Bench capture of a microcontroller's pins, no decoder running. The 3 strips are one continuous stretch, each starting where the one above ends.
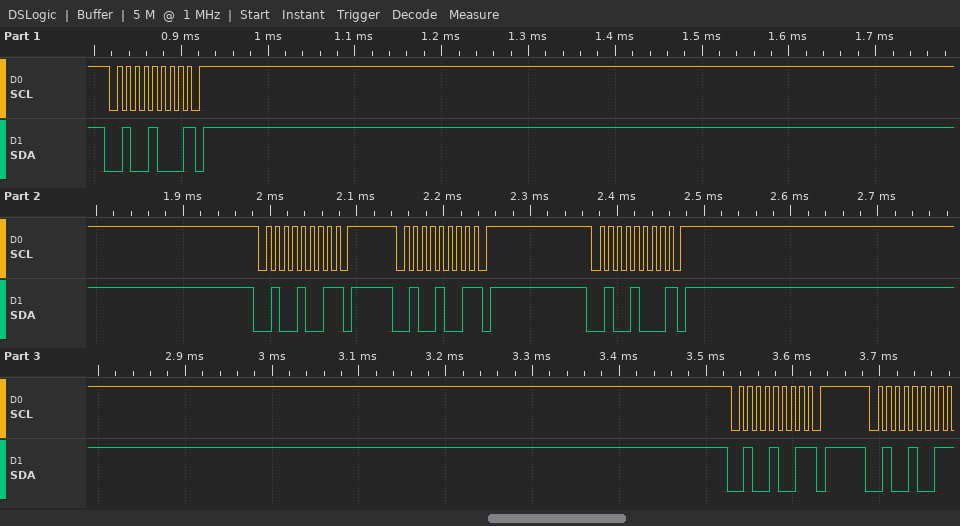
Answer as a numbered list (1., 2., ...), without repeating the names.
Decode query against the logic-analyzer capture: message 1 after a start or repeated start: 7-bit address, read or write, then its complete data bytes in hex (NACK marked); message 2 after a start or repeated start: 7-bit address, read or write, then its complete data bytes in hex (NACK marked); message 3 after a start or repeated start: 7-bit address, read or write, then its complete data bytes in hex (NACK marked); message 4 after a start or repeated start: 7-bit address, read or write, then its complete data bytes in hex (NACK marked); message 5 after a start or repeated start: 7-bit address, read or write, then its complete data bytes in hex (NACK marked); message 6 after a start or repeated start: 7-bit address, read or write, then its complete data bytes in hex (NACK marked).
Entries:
1. 0x24 write NACK
2. 0x24 read NACK
3. 0x24 read NACK
4. 0x24 write NACK
5. 0x24 read NACK
6. 0x24 read NACK
